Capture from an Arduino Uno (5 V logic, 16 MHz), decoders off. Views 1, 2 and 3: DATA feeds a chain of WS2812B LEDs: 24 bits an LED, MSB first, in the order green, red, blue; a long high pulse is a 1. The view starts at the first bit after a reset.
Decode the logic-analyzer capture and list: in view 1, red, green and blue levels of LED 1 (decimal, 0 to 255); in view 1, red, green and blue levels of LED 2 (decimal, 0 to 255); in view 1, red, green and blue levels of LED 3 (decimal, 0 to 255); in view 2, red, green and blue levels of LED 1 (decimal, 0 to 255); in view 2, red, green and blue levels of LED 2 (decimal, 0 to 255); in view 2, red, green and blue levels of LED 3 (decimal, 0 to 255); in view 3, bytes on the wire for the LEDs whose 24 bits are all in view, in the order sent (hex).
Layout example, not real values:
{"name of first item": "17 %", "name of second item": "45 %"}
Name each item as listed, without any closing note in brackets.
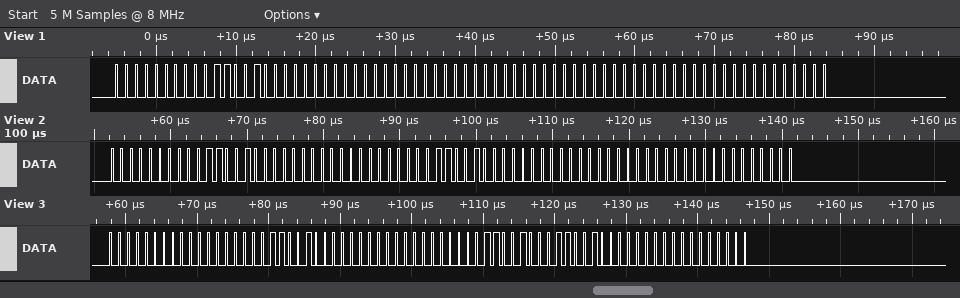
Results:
{"in view 1, red, green and blue levels of LED 1": "50, 0, 0", "in view 1, red, green and blue levels of LED 2": "0, 0, 0", "in view 1, red, green and blue levels of LED 3": "0, 0, 0", "in view 2, red, green and blue levels of LED 1": "50, 0, 0", "in view 2, red, green and blue levels of LED 2": "50, 0, 0", "in view 2, red, green and blue levels of LED 3": "0, 0, 0", "in view 3, bytes on the wire for the LEDs whose 24 bits are all in view, in the order sent": "00 00 32 00 00 32 32 00 00"}
